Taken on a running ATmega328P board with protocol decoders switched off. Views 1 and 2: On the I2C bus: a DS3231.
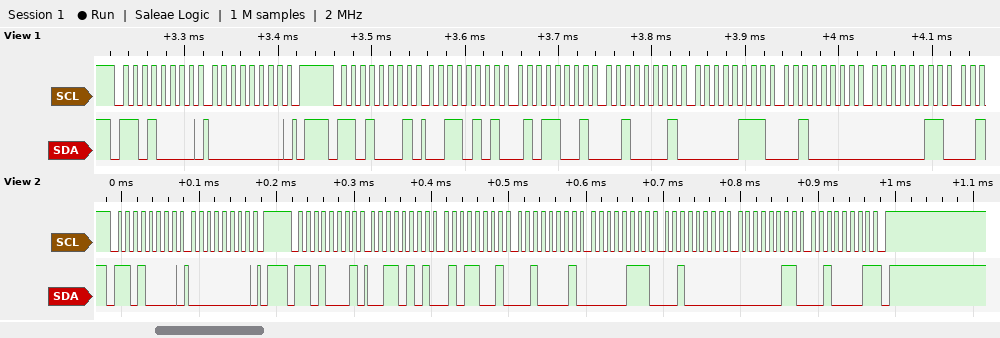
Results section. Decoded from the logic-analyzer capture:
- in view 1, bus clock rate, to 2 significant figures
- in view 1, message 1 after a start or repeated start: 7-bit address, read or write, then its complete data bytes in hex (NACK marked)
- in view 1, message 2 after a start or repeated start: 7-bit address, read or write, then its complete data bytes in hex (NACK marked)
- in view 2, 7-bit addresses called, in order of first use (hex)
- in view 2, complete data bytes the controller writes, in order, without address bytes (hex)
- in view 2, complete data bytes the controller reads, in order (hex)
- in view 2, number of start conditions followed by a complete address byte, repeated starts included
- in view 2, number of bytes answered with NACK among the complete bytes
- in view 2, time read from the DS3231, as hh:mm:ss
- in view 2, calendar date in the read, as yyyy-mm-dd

100 kHz
0x68 write: 00
0x68 read: 35 59 21 07 20 03
0x68
00
35 59 21 07 20 03 21
2
1
21:59:35
2021-03-20
